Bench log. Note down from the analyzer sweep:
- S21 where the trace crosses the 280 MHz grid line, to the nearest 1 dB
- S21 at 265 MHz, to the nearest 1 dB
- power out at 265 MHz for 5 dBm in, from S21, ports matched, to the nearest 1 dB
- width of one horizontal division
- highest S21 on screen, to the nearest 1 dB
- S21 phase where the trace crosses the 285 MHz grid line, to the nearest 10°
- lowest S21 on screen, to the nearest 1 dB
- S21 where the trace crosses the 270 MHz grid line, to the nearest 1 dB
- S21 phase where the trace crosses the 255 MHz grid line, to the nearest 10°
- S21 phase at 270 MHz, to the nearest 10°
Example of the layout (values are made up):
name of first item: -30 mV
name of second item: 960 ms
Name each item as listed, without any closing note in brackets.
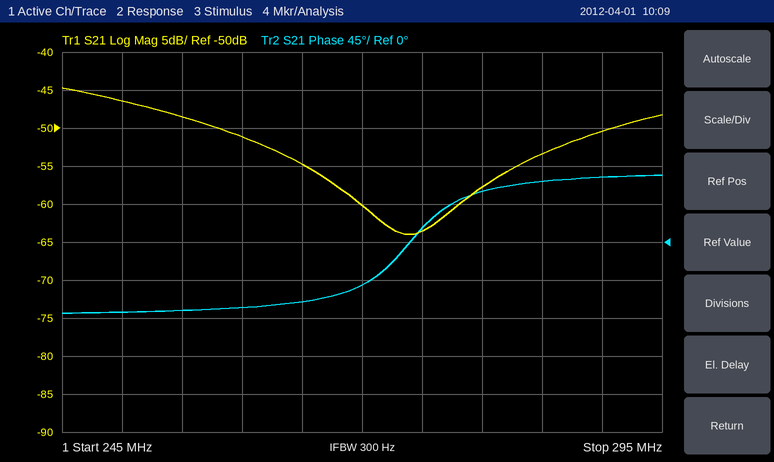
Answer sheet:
S21 where the trace crosses the 280 MHz grid line, to the nearest 1 dB: -58 dB
S21 at 265 MHz, to the nearest 1 dB: -55 dB
power out at 265 MHz for 5 dBm in, from S21, ports matched, to the nearest 1 dB: -50 dBm
width of one horizontal division: 5 MHz
highest S21 on screen, to the nearest 1 dB: -45 dB
S21 phase where the trace crosses the 285 MHz grid line, to the nearest 10°: 70°
lowest S21 on screen, to the nearest 1 dB: -64 dB
S21 where the trace crosses the 270 MHz grid line, to the nearest 1 dB: -60 dB
S21 phase where the trace crosses the 255 MHz grid line, to the nearest 10°: -80°
S21 phase at 270 MHz, to the nearest 10°: -50°
